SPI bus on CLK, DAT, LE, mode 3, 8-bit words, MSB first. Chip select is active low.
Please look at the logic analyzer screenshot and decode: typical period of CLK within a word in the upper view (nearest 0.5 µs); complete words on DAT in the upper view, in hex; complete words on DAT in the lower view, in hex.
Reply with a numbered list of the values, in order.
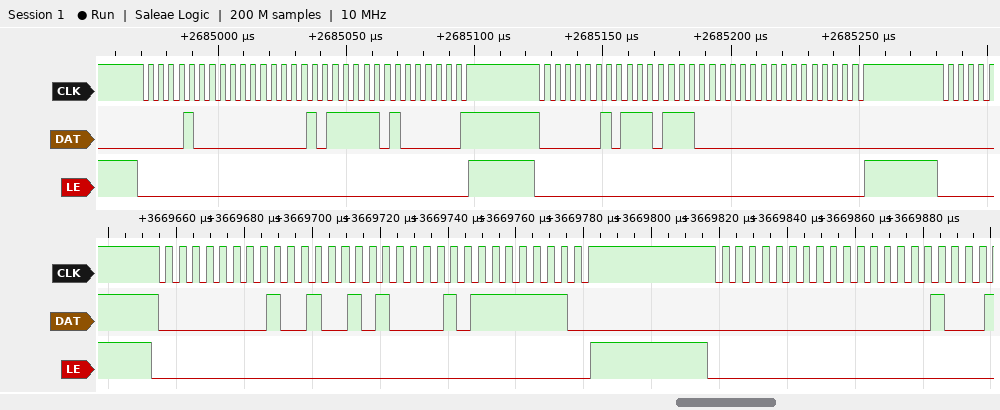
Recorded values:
1. 4 µs
2. 08, 00, BE, 81, 02, EE, 00, 00
3. 00, 92, 85, FC, 00, 00
